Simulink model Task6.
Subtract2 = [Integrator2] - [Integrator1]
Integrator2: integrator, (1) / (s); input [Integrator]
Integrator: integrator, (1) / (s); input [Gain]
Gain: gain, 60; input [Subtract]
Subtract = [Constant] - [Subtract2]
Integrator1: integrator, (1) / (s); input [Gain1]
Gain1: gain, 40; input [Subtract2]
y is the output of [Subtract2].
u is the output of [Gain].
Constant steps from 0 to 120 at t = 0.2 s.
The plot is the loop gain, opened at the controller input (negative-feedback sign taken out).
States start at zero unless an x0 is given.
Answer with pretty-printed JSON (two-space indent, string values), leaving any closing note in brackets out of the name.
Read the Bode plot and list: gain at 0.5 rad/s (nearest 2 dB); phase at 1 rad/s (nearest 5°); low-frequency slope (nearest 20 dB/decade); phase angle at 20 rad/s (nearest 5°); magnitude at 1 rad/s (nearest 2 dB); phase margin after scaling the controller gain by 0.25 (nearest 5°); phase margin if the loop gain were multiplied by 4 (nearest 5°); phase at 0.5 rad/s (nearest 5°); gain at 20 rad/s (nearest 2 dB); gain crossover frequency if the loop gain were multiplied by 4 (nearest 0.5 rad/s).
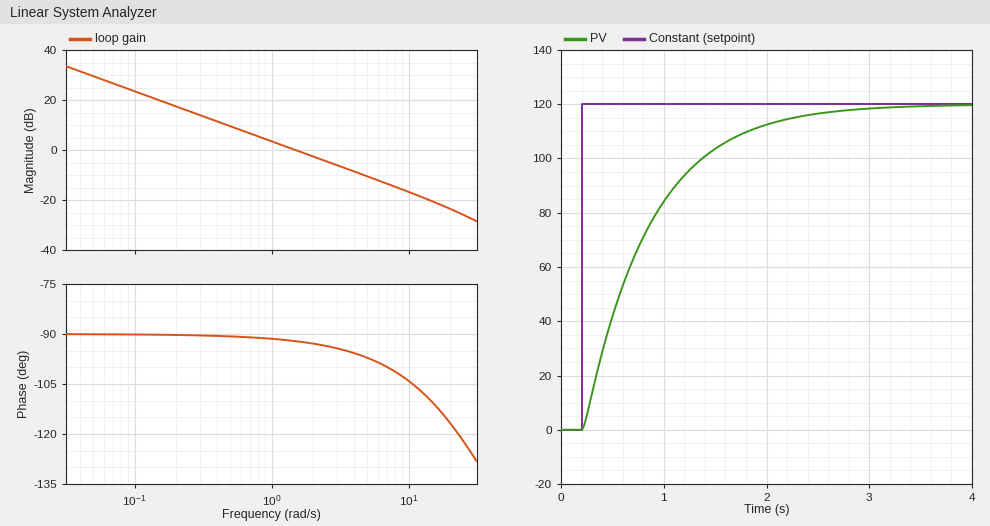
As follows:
{
  "gain at 0.5 rad/s": "10 dB",
  "phase at 1 rad/s": "-90°",
  "low-frequency slope": "-20 dB/decade",
  "phase angle at 20 rad/s": "-115°",
  "magnitude at 1 rad/s": "4 dB",
  "phase margin after scaling the controller gain by 0.25": "90°",
  "phase margin if the loop gain were multiplied by 4": "80°",
  "phase at 0.5 rad/s": "-90°",
  "gain at 20 rad/s": "-24 dB",
  "gain crossover frequency if the loop gain were multiplied by 4": "6.0 rad/s"
}
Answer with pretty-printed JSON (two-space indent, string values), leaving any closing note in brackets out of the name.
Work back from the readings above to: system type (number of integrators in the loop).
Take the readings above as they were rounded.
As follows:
{
  "system type": "1"
}
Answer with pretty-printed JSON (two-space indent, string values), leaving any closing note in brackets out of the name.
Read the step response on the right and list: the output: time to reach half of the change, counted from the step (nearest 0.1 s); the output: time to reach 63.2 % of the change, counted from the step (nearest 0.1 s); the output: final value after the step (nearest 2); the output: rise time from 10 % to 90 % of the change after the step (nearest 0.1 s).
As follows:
{
  "the output: time to reach half of the change, counted from the step": "0.5 s",
  "the output: time to reach 63.2 % of the change, counted from the step": "0.7 s",
  "the output: final value after the step": "120",
  "the output: rise time from 10 % to 90 % of the change after the step": "1.4 s"
}
